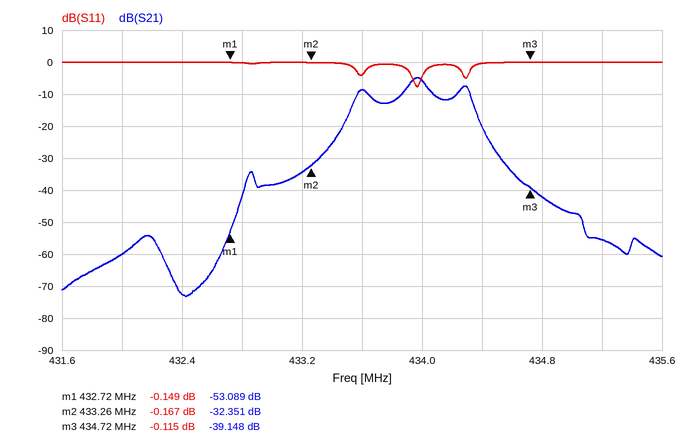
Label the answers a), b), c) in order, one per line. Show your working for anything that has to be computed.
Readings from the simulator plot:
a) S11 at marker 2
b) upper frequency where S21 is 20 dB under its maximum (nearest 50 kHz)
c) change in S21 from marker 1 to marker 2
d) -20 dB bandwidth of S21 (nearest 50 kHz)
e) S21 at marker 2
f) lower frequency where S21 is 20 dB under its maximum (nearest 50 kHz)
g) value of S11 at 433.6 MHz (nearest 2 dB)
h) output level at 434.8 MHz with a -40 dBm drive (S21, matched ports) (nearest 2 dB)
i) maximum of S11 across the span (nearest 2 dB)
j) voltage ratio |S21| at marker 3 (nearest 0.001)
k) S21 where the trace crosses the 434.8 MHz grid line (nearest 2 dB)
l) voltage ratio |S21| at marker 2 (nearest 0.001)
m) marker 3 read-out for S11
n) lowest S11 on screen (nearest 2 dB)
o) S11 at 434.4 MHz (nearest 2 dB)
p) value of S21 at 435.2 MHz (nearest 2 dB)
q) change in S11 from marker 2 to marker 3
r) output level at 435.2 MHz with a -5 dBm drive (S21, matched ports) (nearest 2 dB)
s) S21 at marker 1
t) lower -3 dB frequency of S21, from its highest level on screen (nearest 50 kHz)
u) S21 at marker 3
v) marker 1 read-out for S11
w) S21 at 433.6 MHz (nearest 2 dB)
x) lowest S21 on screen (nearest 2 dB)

a) -0.167 dB
b) 434.45 MHz
c) -32.351 − (-53.089) = 20.738 dB
d) 434.45 MHz − 433.40 MHz = 1.05 MHz
e) -32.351 dB
f) 433.40 MHz
g) -4 dB
h) -40 dBm + (-42 dB) = -82 dBm
i) 0 dB
j) 10^(-39.148/20) ≈ 0.011
k) -42 dB
l) 10^(-32.351/20) ≈ 0.024
m) -0.115 dB
n) -8 dB
o) 0 dB
p) -56 dB
q) -0.115 − (-0.167) = 0.052 dB
r) -5 dBm + (-56 dB) = -60 dBm
s) -53.089 dB
t) 433.90 MHz
u) -39.148 dB
v) -0.149 dB
w) -8 dB
x) -74 dB
